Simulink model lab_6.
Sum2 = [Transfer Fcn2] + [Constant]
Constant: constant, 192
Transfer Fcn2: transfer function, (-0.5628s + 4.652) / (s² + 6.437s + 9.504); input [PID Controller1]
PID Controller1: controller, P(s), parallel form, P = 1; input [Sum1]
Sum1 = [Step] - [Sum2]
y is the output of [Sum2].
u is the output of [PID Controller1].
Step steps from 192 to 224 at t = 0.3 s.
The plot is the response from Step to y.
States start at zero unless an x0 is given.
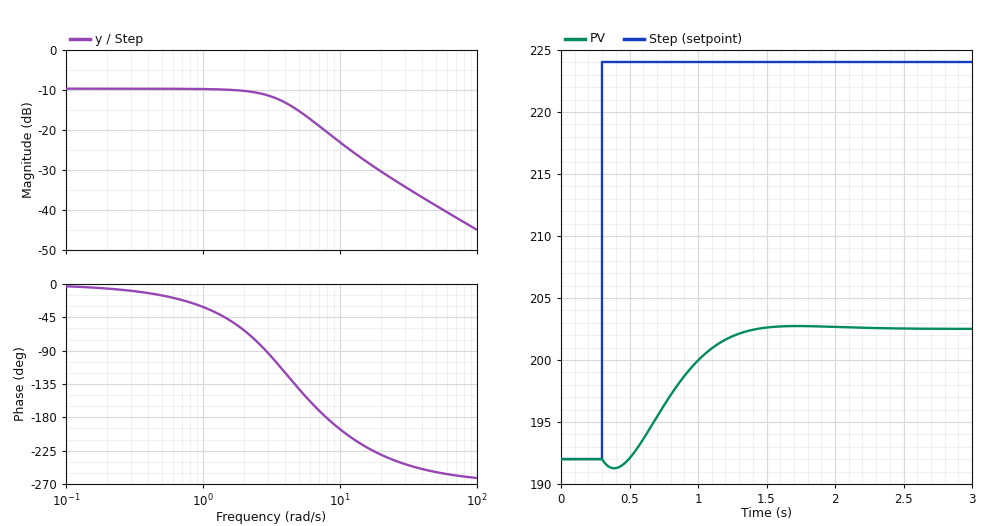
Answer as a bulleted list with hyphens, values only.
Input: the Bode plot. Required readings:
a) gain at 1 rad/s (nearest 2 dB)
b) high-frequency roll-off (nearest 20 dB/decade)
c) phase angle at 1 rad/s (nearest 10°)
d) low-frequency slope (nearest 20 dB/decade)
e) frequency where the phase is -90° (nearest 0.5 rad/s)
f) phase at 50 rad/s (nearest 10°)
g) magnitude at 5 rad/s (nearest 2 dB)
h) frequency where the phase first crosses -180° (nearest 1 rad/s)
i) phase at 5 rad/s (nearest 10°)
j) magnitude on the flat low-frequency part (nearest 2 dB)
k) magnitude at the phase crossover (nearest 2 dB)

- -10 dB
- -20 dB/decade
- -30°
- 0 dB/decade
- 3.0 rad/s
- -250°
- -16 dB
- 8 rad/s
- -140°
- -10 dB
- -20 dB
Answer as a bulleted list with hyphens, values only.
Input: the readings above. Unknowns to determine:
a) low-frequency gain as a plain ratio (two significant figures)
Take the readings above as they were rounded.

- 0.32
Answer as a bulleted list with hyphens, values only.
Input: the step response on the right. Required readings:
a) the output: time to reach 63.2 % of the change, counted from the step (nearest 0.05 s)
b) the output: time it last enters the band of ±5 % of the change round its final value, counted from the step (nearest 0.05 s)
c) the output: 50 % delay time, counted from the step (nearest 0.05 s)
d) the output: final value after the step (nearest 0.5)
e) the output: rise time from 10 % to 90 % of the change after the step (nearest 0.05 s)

- 0.60 s
- 0.95 s
- 0.50 s
- 202.5
- 0.60 s
